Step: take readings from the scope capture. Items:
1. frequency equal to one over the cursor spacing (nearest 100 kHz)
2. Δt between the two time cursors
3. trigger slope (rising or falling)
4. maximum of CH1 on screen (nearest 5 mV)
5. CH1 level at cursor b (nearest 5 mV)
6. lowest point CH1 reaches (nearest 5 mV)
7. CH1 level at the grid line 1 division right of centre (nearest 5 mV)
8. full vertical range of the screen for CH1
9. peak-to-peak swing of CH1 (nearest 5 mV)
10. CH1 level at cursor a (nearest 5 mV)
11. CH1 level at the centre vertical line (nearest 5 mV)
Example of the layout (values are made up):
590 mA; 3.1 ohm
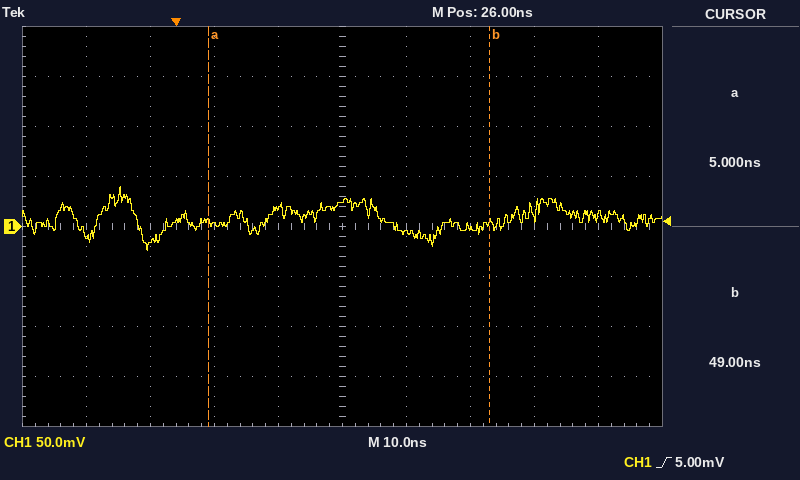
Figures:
22.7 MHz; 44 ns; rising; 40 mV; 5 mV; -25 mV; -5 mV; 400 mV; 65 mV; 5 mV; 25 mV
